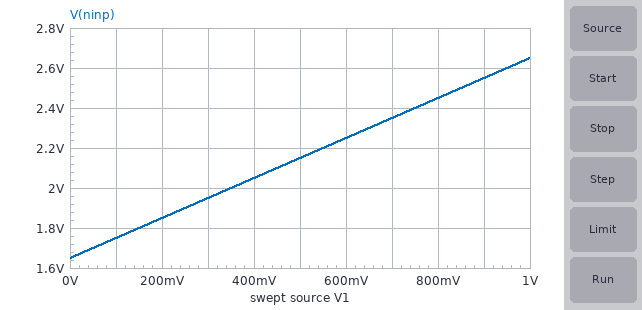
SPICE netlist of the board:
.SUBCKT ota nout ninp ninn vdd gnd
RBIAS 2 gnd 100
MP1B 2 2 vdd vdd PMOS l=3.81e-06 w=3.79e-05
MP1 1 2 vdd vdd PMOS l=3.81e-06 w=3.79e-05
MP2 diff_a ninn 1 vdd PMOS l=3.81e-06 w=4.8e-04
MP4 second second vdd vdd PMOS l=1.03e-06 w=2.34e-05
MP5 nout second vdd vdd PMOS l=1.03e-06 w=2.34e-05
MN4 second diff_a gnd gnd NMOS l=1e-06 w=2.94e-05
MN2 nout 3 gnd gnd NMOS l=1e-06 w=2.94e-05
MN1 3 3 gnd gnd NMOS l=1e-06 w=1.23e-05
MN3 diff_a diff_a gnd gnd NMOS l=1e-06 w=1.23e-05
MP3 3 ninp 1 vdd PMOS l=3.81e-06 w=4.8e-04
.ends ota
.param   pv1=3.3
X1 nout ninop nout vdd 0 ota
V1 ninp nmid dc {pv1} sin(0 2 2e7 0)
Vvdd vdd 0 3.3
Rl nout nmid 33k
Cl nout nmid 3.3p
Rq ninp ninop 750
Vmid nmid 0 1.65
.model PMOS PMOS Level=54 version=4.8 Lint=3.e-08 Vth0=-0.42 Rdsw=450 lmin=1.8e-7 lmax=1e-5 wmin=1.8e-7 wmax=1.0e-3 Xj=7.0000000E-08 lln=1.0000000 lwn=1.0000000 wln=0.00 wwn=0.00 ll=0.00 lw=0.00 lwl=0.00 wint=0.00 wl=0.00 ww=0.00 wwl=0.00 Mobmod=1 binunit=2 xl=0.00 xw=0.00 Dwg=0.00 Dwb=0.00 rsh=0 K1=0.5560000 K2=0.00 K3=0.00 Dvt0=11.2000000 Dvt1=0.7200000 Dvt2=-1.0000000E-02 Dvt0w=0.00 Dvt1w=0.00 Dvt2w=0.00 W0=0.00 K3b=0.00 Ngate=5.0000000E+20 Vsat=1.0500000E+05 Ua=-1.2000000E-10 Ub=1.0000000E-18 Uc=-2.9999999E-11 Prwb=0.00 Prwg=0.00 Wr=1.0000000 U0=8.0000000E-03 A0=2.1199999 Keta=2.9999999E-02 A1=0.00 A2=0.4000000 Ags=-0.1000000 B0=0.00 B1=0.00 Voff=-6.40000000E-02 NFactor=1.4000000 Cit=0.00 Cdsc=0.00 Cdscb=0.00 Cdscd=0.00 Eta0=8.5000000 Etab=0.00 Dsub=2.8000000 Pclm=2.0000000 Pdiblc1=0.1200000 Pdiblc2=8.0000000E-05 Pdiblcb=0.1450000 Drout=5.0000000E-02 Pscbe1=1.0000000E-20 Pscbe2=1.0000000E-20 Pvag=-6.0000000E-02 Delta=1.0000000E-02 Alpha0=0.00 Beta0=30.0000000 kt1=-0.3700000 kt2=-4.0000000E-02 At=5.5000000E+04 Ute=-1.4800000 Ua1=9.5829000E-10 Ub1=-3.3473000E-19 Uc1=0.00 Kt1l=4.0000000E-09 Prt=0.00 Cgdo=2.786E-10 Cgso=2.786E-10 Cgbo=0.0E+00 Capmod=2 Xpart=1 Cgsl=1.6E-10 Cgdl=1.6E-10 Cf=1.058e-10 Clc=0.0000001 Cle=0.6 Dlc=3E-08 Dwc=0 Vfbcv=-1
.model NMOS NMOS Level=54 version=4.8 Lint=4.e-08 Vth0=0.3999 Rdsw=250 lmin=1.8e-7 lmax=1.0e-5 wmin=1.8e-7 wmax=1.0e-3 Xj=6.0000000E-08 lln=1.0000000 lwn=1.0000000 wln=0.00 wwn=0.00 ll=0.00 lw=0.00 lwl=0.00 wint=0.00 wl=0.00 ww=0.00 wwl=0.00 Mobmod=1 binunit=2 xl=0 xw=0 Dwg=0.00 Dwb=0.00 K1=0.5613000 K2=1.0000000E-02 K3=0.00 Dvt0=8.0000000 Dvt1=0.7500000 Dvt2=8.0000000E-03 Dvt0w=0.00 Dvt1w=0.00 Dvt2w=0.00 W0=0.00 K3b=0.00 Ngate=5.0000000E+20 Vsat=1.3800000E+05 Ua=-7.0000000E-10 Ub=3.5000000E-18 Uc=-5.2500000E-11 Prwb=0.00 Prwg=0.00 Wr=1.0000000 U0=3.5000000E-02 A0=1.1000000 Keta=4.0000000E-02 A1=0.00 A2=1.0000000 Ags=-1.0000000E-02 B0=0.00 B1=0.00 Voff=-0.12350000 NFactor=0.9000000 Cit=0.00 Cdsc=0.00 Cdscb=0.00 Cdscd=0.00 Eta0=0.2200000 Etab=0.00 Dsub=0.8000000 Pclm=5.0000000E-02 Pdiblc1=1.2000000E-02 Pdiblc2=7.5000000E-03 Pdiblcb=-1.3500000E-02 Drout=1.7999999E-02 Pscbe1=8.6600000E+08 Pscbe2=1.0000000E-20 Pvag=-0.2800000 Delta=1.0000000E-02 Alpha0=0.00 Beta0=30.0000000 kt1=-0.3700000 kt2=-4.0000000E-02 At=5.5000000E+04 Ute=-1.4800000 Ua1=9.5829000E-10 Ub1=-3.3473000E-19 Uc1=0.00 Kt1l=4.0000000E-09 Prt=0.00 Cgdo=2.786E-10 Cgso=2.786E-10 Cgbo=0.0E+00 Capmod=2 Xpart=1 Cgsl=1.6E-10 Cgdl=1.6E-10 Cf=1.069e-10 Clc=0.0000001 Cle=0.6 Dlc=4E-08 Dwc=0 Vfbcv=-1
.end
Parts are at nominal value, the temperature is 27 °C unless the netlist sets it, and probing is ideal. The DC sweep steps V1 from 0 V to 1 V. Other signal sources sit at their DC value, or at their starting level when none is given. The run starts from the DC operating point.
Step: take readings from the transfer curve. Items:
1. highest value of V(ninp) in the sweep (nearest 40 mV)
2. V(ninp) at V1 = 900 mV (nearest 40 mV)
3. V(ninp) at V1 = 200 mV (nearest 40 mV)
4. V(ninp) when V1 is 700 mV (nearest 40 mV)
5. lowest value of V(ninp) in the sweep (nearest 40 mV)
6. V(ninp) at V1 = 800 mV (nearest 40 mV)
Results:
2.64 V
2.56 V
1.84 V
2.36 V
1.64 V
2.44 V
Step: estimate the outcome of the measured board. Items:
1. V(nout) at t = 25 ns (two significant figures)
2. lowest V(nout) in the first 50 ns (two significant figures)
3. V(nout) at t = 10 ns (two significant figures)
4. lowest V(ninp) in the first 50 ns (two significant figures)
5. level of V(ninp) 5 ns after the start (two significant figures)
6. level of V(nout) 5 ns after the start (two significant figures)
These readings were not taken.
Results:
2.7 V
180 mV
2.4 V
-350 mV
2.8 V
1.9 V
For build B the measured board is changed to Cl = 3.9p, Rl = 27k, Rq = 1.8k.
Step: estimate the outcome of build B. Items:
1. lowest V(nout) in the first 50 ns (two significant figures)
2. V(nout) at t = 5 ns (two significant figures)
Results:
190 mV
1.8 V
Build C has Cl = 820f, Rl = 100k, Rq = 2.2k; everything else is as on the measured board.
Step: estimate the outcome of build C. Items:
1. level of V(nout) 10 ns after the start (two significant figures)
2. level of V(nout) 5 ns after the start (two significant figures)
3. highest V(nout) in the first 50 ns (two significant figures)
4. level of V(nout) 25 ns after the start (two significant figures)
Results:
2.2 V
1.8 V
2.8 V
2.8 V
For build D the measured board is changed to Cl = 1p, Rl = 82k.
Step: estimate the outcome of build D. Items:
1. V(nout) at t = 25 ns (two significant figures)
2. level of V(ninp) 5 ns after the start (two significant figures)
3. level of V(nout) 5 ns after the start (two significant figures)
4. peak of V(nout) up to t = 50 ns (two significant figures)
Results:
2.8 V
2.8 V
2.0 V
2.9 V
